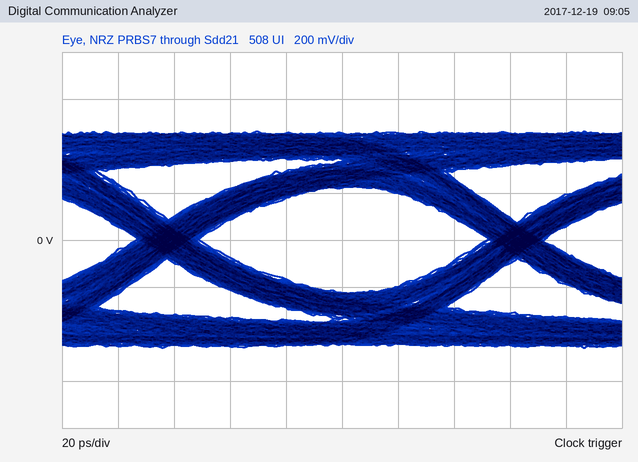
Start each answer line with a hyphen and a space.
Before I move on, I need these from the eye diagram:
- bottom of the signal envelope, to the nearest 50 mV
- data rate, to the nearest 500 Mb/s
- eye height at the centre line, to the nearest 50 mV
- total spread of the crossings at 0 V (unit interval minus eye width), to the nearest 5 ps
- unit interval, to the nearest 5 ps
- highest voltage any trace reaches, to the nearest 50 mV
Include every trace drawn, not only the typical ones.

- -450 mV
- 8.0 Gb/s
- 450 mV
- 20 ps
- 125 ps
- 450 mV
